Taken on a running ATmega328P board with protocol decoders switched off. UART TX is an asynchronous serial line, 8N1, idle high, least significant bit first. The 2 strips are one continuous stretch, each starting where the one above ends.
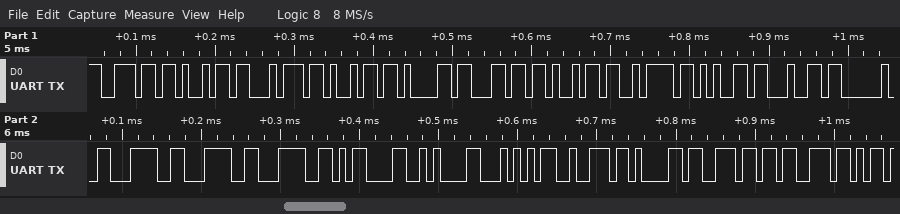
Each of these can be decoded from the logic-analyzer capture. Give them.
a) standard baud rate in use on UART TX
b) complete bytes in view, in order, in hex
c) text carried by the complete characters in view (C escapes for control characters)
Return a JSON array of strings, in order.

["115200 baud", "6E 69 74 69 61 6C 69 7A 65 64 20 3C 3C 3C 0D 0A 54 72 61 6E 73", "\"nitialized <<<\\r\\nTrans\""]
